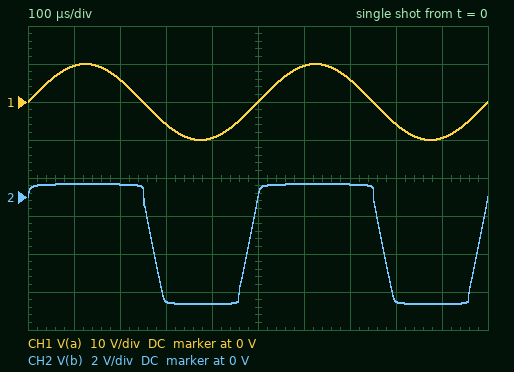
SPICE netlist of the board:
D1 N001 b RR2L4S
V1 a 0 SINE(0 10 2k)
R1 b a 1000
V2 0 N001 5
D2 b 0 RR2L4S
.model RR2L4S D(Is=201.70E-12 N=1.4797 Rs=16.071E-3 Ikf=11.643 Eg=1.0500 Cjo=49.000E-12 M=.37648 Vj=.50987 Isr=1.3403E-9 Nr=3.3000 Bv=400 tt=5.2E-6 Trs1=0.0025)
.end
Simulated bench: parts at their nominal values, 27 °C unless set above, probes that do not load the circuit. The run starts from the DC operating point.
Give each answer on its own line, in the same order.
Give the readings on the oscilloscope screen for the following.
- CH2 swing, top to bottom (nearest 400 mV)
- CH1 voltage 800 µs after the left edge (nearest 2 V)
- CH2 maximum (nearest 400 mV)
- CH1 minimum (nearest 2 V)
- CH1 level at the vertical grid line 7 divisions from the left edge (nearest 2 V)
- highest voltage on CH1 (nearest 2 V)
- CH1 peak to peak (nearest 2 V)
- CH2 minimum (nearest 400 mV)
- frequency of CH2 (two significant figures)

6.4 V
-6 V
800 mV
-10 V
6 V
10 V
20 V
-5.6 V
2.0 kHz
